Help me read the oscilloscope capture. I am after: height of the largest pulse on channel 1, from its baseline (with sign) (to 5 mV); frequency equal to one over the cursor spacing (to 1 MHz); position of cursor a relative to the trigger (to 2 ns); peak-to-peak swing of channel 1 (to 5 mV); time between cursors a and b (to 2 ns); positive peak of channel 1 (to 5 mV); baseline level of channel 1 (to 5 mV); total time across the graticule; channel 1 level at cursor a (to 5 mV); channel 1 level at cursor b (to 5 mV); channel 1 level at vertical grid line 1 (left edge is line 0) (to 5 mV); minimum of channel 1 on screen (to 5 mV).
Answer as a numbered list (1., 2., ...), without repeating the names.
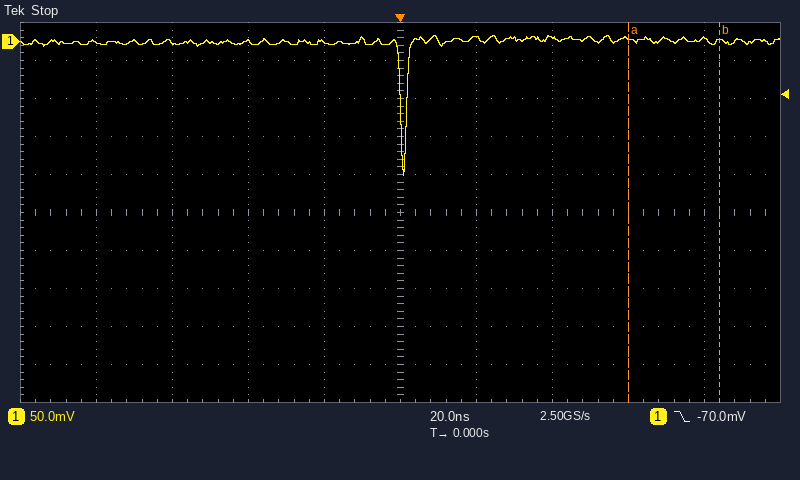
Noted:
1. -175 mV
2. 42 MHz
3. +60 ns
4. 185 mV
5. 24 ns
6. 10 mV
7. 0 mV
8. 200 ns
9. 5 mV
10. 0 mV
11. 0 mV
12. -175 mV
